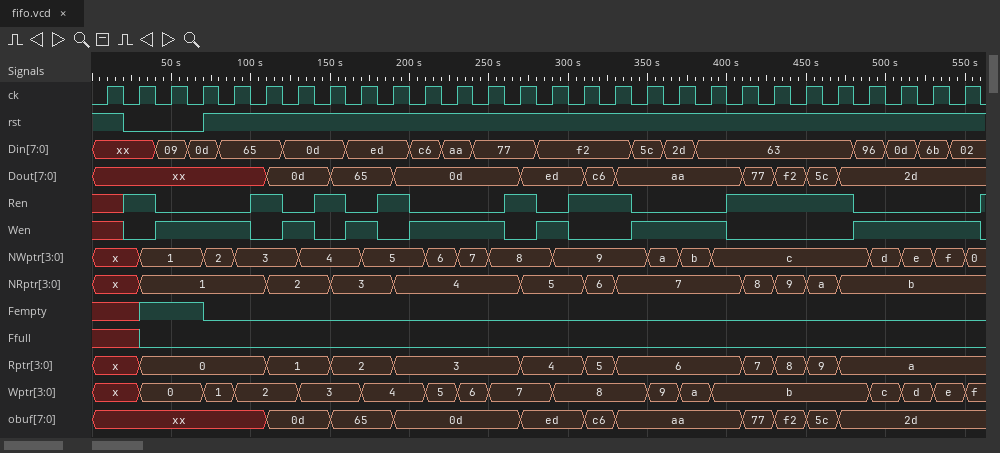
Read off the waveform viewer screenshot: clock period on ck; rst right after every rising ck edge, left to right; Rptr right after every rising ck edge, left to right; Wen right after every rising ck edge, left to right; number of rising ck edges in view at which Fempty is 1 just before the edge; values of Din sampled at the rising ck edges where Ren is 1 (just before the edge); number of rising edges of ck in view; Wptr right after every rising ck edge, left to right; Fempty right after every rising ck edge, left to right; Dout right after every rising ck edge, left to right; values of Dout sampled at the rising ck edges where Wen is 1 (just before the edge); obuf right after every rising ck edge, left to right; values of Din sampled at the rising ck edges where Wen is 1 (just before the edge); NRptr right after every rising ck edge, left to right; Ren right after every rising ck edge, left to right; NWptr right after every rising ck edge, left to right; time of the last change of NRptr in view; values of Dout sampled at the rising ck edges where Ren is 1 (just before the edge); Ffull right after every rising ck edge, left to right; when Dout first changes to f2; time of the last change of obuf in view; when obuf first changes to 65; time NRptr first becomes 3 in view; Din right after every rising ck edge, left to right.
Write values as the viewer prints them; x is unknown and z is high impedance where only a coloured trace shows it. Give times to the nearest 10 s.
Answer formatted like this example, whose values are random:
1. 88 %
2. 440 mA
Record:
1. 20 s
2. 1 0 0 1 1 1 1 1 1 1 1 1 1 1 1 1 1 1 1 1 1 1 1 1 1 1 1 1
3. x, 0, 0, 0, 0, 1, 1, 2, 2, 3, 3, 3, 3, 4, 4, 5, 6, 6, 6, 6, 7, 8, 9, a, a, a, a, a
4. x 0 1 1 1 0 1 0 1 0 1 1 1 0 1 0 0 1 1 1 0 0 0 0 1 1 1 1
5. 2
6. xx, 65, 0d, ed, 77, f2, f2, 63, 63, 63, 63
7. 28
8. x, 0, 0, 1, 2, 2, 3, 3, 4, 4, 5, 6, 7, 7, 8, 8, 8, 9, a, b, b, b, b, b, c, d, e, f
9. x 1 1 0 0 0 0 0 0 0 0 0 0 0 0 0 0 0 0 0 0 0 0 0 0 0 0 0
10. xx, xx, xx, xx, xx, 0d, 0d, 65, 65, 0d, 0d, 0d, 0d, ed, ed, c6, aa, aa, aa, aa, 77, f2, 5c, 2d, 2d, 2d, 2d, 2d
11. xx, xx, xx, 0d, 65, 0d, 0d, 0d, ed, aa, aa, aa, 2d, 2d, 2d, 2d
12. xx, xx, xx, xx, xx, 0d, 0d, 65, 65, 0d, 0d, 0d, 0d, ed, ed, c6, aa, aa, aa, aa, 77, f2, 5c, 2d, 2d, 2d, 2d, 2d
13. 09, 0d, 65, 0d, ed, c6, aa, 77, f2, 5c, 2d, 63, 96, 0d, 6b, 02
14. x, 1, 1, 1, 1, 2, 2, 3, 3, 4, 4, 4, 4, 5, 5, 6, 7, 7, 7, 7, 8, 9, a, b, b, b, b, b
15. x 1 0 0 0 1 0 1 0 1 0 0 0 1 0 1 1 0 0 0 1 1 1 1 0 0 0 0
16. x, 1, 1, 2, 3, 3, 4, 4, 5, 5, 6, 7, 8, 8, 9, 9, 9, a, b, c, c, c, c, c, d, e, f, 0
17. 470 s
18. xx, xx, 0d, 65, 0d, ed, c6, aa, 77, f2, 5c
19. x 0 0 0 0 0 0 0 0 0 0 0 0 0 0 0 0 0 0 0 0 0 0 0 0 0 0 0
20. 430 s
21. 470 s
22. 150 s
23. 150 s
24. xx, xx, 09, 0d, 65, 65, 0d, 0d, ed, ed, c6, aa, 77, 77, f2, f2, f2, 5c, 2d, 63, 63, 63, 63, 63, 96, 0d, 6b, 02
